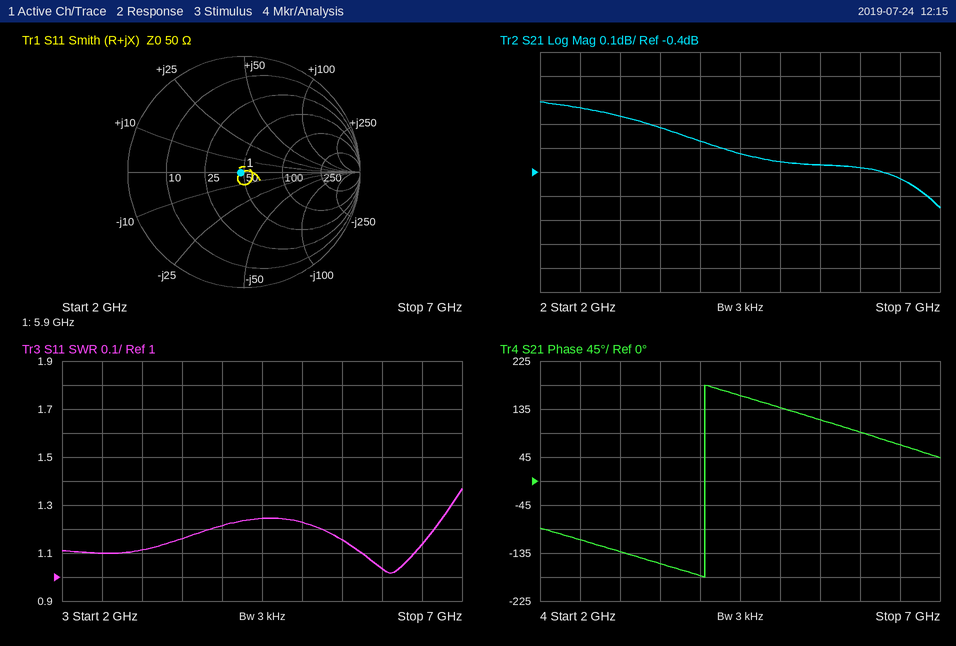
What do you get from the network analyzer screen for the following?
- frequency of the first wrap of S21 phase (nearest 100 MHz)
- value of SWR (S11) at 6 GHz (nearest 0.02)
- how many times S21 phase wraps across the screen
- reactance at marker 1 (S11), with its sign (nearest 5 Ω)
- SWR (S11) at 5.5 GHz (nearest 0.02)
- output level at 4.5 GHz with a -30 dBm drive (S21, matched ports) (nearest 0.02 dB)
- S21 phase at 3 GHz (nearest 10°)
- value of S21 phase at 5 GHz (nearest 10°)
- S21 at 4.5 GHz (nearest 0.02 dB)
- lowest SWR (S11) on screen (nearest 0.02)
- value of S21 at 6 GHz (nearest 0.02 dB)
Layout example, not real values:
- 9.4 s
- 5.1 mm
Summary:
- 4.1 GHz
- 1.04
- 1
- 0 Ω
- 1.16
- -30.32 dBm
- -130°
- 140°
- -0.32 dB
- 1.02
- -0.38 dB
